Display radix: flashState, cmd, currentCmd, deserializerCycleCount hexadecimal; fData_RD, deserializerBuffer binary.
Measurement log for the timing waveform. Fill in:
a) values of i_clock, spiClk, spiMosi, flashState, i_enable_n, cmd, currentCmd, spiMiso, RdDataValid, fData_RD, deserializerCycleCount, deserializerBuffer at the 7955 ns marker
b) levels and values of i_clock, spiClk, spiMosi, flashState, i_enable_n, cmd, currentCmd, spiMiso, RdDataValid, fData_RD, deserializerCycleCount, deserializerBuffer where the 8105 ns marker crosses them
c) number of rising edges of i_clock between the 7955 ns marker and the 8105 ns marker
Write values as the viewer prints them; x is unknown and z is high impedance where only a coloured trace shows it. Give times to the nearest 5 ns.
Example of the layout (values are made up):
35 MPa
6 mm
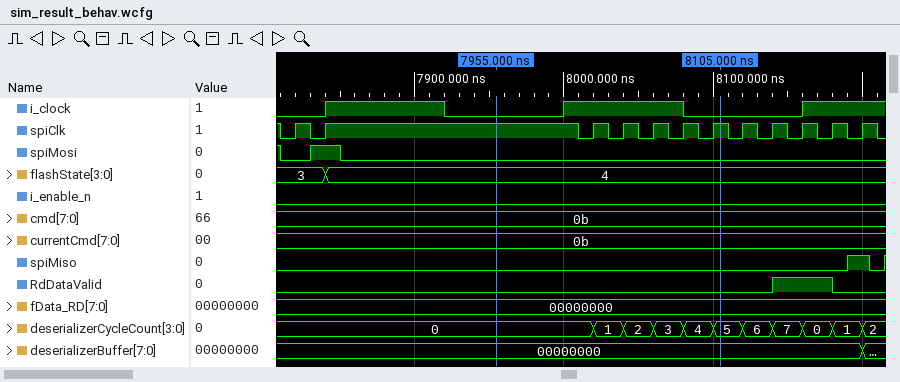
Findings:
i_clock=0, spiClk=1, spiMosi=0, flashState=4, i_enable_n=0, cmd=0b, currentCmd=0b, spiMiso=0, RdDataValid=0, fData_RD=00000000, deserializerCycleCount=0, deserializerBuffer=00000000
i_clock=0, spiClk=1, spiMosi=0, flashState=4, i_enable_n=0, cmd=0b, currentCmd=0b, spiMiso=0, RdDataValid=0, fData_RD=00000000, deserializerCycleCount=5, deserializerBuffer=00000000
1
